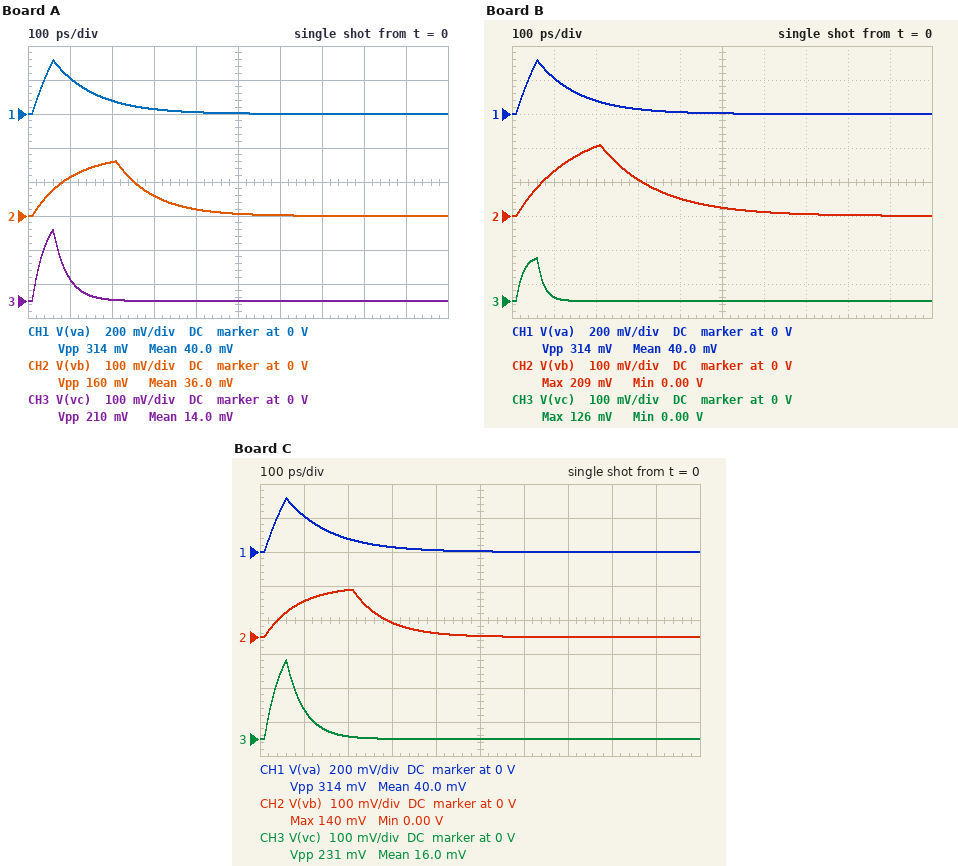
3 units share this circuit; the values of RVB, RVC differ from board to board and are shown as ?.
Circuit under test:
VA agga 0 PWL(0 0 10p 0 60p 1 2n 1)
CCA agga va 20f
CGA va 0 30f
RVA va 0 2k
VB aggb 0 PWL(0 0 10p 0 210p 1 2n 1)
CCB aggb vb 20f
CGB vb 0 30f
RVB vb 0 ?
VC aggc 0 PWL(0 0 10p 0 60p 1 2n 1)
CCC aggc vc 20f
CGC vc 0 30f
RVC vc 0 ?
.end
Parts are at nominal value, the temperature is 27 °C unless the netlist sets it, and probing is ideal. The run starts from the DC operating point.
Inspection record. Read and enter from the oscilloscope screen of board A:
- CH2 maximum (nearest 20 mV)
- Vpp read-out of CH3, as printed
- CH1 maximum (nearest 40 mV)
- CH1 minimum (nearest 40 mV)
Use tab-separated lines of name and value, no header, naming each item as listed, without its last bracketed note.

CH2 maximum	160 mV
Vpp read-out of CH3, as printed	210 mV
CH1 maximum	320 mV
CH1 minimum	0 V
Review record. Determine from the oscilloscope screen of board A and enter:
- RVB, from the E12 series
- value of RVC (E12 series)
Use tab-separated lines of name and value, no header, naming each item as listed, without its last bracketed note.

RVB, from the E12 series	1.8 kΩ
value of RVC	680 Ω
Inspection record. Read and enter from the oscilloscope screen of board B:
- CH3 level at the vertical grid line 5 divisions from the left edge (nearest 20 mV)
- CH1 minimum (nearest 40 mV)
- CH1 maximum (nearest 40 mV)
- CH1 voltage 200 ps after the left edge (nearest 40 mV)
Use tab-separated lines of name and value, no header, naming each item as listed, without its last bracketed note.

CH3 level at the vertical grid line 5 divisions from the left edge	0 V
CH1 minimum	0 V
CH1 maximum	320 mV
CH1 voltage 200 ps after the left edge	80 mV
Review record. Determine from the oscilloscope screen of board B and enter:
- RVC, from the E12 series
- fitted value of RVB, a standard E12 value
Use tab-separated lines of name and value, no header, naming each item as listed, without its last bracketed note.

RVC, from the E12 series	330 Ω
fitted value of RVB, a standard E12 value	2.7 kΩ
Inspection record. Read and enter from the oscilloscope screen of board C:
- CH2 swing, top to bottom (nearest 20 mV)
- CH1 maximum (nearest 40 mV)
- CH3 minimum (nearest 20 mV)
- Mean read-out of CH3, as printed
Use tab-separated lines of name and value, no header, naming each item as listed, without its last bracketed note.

CH2 swing, top to bottom	140 mV
CH1 maximum	320 mV
CH3 minimum	0 V
Mean read-out of CH3, as printed	16.0 mV
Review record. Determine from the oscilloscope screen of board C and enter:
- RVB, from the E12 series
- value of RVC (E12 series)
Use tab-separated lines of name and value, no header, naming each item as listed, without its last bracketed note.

RVB, from the E12 series	1.5 kΩ
value of RVC	820 Ω
